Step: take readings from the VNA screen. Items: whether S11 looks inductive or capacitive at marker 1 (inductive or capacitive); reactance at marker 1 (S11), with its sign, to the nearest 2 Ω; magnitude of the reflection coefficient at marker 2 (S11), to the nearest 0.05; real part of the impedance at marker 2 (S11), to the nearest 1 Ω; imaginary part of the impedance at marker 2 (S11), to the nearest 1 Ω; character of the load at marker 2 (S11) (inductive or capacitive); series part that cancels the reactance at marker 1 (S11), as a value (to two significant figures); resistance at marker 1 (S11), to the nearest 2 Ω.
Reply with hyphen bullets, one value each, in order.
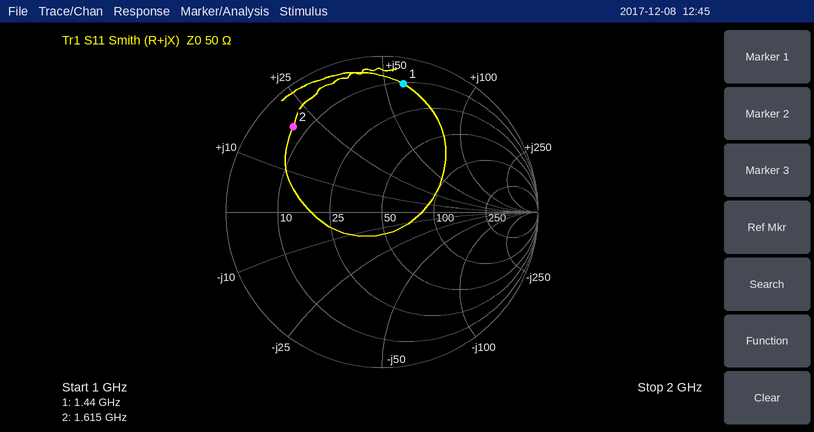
- inductive
- +58 Ω
- 0.80
- 7 Ω
- +20 Ω
- inductive
- 1.9 pF
- 10 Ω
